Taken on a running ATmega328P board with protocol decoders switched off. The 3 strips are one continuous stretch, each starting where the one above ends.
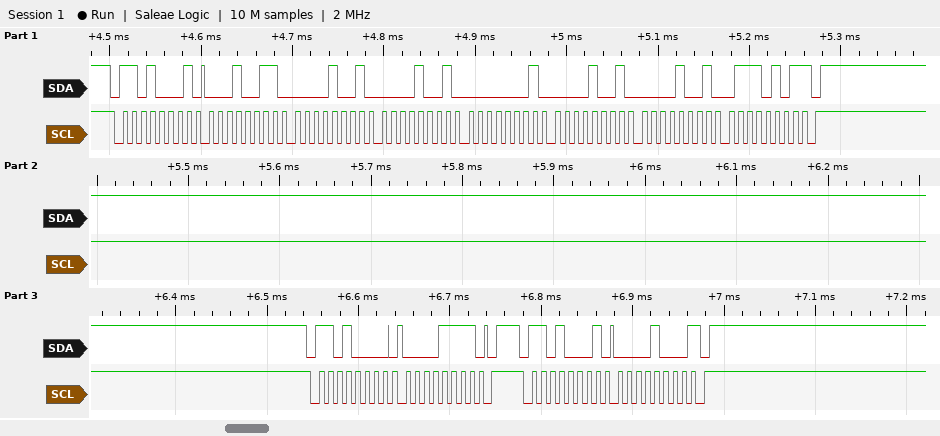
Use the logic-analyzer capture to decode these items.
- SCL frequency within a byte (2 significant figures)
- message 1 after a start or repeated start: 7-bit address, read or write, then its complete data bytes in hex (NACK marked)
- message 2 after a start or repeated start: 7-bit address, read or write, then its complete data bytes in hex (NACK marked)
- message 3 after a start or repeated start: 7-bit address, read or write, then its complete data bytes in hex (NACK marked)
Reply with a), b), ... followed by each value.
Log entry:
a) 100 kHz
b) 0x68 read: 13 09 09 01 09 09 75 NACK
c) 0x68 write: 0F
d) 0x68 read: 08 NACK
